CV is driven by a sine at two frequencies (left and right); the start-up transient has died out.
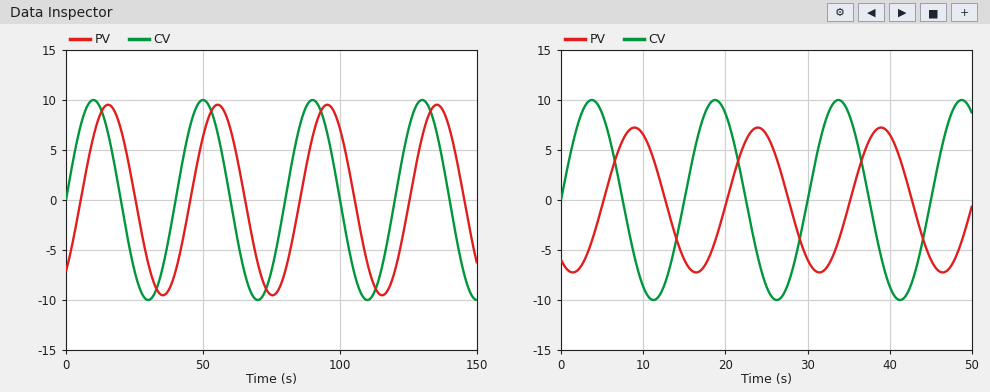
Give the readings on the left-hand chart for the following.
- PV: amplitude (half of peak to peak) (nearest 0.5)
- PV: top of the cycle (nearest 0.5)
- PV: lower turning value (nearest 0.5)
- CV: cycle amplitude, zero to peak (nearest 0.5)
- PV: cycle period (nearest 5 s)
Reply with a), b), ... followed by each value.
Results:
a) 9.5
b) 9.5
c) -9.5
d) 10.0
e) 40 s
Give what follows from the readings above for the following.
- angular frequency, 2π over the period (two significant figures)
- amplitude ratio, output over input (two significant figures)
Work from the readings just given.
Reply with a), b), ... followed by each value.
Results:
a) 0.16 rad/s
b) 0.95
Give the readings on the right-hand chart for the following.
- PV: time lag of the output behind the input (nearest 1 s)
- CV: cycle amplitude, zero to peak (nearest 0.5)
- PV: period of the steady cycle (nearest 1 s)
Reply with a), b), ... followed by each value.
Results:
a) 5 s
b) 10.0
c) 15 s
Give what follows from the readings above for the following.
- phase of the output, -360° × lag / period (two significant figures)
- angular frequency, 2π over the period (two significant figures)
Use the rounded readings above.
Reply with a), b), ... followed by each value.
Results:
a) -120°
b) 0.42 rad/s
